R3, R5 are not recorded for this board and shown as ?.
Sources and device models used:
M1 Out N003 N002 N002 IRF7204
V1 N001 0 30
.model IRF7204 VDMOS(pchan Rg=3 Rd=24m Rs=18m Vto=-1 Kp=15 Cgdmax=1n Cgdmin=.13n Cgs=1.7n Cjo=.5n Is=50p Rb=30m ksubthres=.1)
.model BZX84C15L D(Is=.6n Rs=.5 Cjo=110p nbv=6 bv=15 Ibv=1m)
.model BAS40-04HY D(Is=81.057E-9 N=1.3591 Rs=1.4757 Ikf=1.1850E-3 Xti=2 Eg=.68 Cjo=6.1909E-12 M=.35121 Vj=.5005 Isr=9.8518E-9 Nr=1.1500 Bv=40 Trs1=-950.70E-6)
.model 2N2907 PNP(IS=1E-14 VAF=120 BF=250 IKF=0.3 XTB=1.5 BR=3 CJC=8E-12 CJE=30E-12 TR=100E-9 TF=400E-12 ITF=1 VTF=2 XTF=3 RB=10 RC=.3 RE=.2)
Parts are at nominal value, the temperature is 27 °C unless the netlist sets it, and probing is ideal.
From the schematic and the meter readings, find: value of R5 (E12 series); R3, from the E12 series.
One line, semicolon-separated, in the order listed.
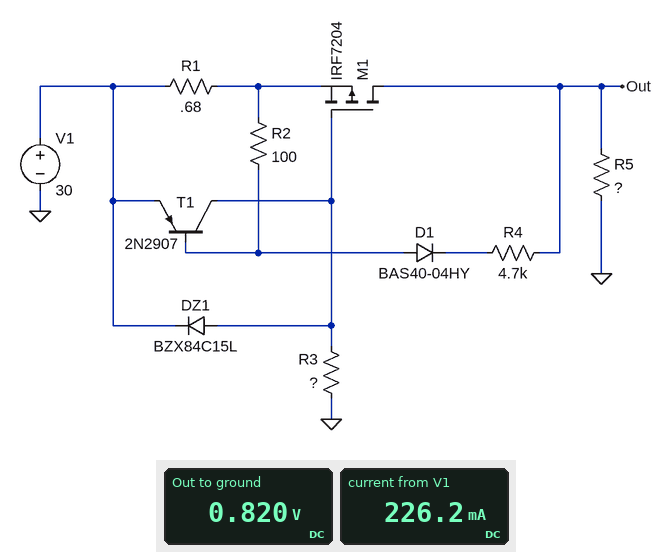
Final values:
3.9 Ω; 1.8 kΩ
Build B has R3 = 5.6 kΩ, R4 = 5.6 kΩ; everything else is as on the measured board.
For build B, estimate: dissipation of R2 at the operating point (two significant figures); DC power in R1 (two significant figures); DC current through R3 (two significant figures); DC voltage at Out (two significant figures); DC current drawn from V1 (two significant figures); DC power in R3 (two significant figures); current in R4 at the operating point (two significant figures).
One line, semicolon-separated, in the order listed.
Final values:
2.4 mW; 63 mW; 5.1 mA; 1.2 V; 310 mA; 150 mW; 4.9 mA
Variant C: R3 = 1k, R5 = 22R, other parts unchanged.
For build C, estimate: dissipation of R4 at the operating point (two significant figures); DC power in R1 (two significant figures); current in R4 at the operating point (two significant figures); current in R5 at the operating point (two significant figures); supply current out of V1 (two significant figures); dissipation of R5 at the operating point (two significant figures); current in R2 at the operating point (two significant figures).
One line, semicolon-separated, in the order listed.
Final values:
38 mW; 340 mW; 2.8 mA; 700 mA; 730 mA; 11 W; 2.7 mA
